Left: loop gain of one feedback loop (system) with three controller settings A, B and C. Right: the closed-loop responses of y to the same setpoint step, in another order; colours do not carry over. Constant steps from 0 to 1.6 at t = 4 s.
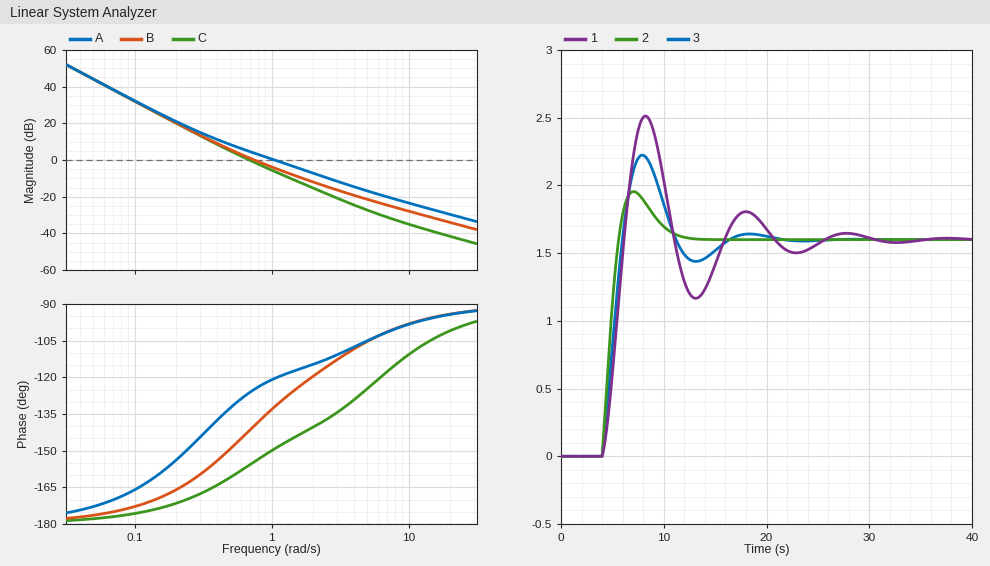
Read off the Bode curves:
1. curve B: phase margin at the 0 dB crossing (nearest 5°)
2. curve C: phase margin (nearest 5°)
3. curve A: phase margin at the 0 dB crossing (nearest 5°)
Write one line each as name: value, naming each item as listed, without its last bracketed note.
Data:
curve B: phase margin at the 0 dB crossing: 40°
curve C: phase margin: 25°
curve A: phase margin at the 0 dB crossing: 60°
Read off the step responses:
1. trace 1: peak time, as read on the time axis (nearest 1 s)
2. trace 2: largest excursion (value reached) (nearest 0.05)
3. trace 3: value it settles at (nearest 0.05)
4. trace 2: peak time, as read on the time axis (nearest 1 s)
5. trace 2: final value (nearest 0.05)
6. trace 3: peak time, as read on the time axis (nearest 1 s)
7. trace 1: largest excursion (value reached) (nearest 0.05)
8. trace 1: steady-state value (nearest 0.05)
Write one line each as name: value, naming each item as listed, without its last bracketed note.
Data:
trace 1: peak time, as read on the time axis: 8 s
trace 2: largest excursion (value reached): 1.95
trace 3: value it settles at: 1.60
trace 2: peak time, as read on the time axis: 7 s
trace 2: final value: 1.60
trace 3: peak time, as read on the time axis: 8 s
trace 1: largest excursion (value reached): 2.50
trace 1: steady-state value: 1.60
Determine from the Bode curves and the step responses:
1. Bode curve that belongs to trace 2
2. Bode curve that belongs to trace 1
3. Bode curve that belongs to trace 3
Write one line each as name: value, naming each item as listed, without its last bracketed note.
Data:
Bode curve that belongs to trace 2: A
Bode curve that belongs to trace 1: C
Bode curve that belongs to trace 3: B
